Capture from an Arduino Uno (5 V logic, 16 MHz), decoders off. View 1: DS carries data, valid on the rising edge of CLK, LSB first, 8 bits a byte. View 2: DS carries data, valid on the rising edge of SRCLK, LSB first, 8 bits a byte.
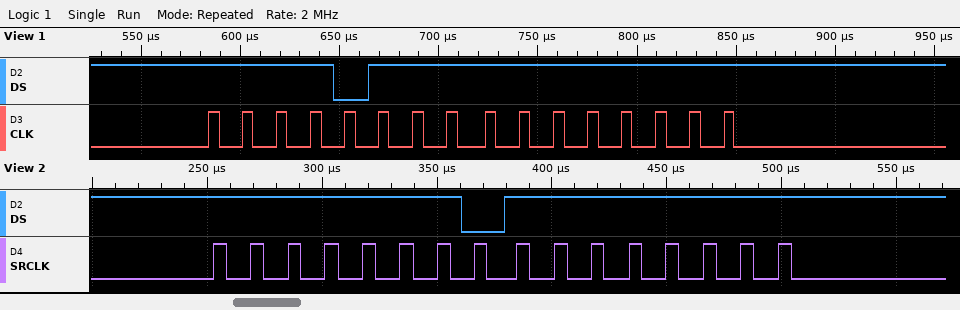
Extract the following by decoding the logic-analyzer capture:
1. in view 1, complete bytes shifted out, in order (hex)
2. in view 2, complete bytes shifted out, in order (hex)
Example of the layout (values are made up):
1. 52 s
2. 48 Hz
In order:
1. EF FF
2. 7F FF
